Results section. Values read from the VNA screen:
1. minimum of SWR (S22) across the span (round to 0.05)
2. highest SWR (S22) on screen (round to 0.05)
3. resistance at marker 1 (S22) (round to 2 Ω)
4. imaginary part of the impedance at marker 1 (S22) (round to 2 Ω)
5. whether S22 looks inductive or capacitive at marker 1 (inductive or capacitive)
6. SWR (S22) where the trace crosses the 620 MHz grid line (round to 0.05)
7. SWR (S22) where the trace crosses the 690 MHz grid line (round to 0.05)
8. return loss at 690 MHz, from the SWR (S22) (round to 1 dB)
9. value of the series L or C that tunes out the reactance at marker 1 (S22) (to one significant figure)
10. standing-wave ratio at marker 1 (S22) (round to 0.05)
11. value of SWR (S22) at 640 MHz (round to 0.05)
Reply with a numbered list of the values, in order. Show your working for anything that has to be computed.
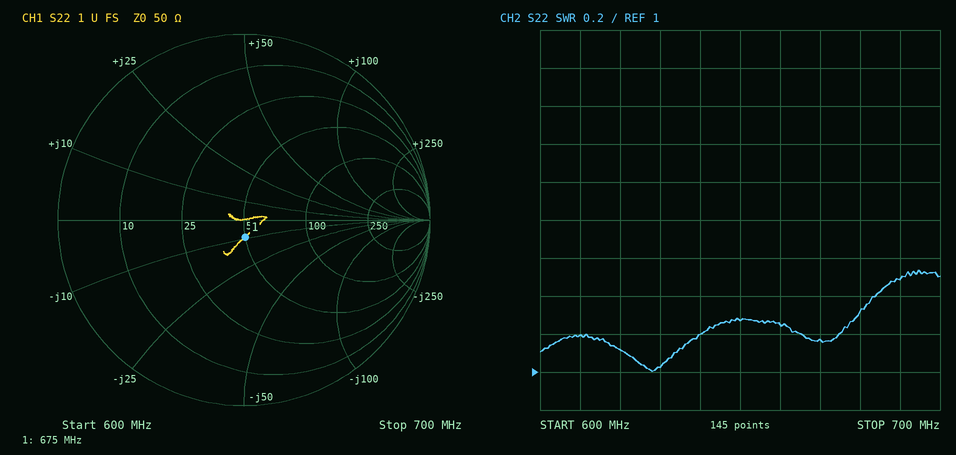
1. 1.00
2. 1.55
3. 50 Ω
4. -10 Ω
5. capacitive
6. 1.10
7. 1.50
8. −20 log10((1.5 − 1)/(1.5 + 1)) ≈ 14 dB
9. L = 10 Ω/(2π × 675 MHz) ≈ 2 nH
10. 1.20
11. 1.20
